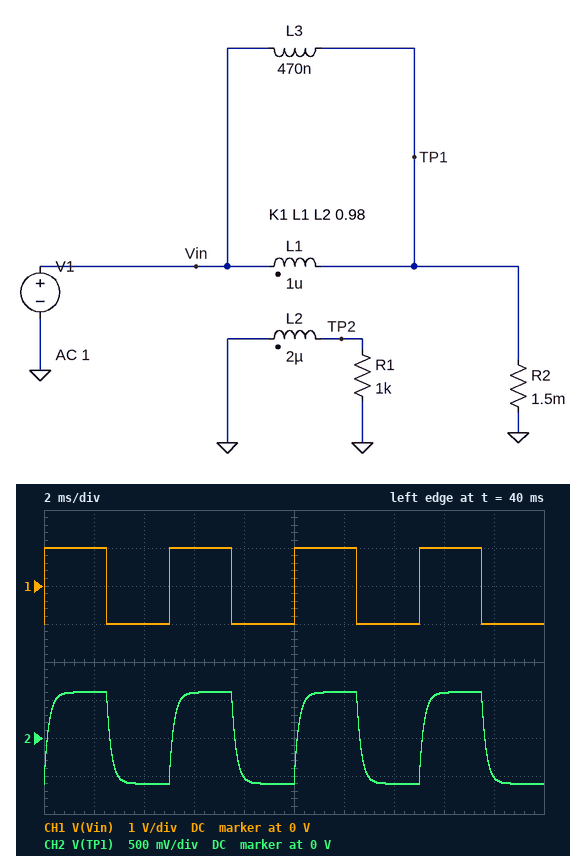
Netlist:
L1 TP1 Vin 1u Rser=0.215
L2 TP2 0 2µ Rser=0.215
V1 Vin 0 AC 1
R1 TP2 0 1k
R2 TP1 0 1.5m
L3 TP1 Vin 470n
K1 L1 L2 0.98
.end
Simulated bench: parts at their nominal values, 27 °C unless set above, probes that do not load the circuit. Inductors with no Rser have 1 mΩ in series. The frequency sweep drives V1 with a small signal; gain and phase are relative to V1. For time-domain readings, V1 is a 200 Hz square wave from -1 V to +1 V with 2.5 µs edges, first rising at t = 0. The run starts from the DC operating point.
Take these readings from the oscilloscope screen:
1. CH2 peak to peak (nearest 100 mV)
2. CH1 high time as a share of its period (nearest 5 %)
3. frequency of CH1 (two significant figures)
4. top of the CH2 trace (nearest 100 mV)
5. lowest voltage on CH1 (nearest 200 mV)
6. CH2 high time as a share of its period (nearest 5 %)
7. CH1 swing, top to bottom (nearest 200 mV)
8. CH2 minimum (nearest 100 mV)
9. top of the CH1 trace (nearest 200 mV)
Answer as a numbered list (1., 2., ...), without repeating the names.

1. 1.2 V
2. 50 %
3. 200 Hz
4. 600 mV
5. -1.0 V
6. 50 %
7. 2.0 V
8. -600 mV
9. 1.0 V
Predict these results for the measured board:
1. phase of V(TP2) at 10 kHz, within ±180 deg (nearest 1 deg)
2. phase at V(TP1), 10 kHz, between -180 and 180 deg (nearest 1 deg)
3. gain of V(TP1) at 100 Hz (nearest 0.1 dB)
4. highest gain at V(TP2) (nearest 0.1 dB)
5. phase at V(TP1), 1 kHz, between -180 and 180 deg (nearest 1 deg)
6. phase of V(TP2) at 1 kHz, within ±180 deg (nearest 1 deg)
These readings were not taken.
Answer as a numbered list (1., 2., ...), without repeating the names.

1. -103 deg
2. -78 deg
3. -4.5 dB
4. 2.8 dB
5. -49 deg
6. -70 deg
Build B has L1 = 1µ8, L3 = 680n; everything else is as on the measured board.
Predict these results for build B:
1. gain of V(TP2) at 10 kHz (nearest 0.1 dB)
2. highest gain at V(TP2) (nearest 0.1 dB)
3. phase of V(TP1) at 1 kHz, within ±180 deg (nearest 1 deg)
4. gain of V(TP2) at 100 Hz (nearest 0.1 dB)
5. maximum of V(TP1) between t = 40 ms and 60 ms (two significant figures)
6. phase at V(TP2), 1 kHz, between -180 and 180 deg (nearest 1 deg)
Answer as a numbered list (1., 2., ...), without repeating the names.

1. -6.4 dB
2. 0.3 dB
3. -59 deg
4. -52.7 dB
5. 600 mV
6. -76 deg
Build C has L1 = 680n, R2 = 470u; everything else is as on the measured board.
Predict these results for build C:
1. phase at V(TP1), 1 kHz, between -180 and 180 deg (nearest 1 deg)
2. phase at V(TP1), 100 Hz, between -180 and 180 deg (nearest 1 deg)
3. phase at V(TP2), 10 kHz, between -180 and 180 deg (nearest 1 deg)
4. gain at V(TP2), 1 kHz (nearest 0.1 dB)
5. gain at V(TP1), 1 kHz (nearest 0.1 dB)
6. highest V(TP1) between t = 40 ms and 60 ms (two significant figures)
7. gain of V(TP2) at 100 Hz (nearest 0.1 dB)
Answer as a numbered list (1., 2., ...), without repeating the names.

1. -63 deg
2. -11 deg
3. -100 deg
4. -30.0 dB
5. -16.9 dB
6. 320 mV
7. -52.7 dB
